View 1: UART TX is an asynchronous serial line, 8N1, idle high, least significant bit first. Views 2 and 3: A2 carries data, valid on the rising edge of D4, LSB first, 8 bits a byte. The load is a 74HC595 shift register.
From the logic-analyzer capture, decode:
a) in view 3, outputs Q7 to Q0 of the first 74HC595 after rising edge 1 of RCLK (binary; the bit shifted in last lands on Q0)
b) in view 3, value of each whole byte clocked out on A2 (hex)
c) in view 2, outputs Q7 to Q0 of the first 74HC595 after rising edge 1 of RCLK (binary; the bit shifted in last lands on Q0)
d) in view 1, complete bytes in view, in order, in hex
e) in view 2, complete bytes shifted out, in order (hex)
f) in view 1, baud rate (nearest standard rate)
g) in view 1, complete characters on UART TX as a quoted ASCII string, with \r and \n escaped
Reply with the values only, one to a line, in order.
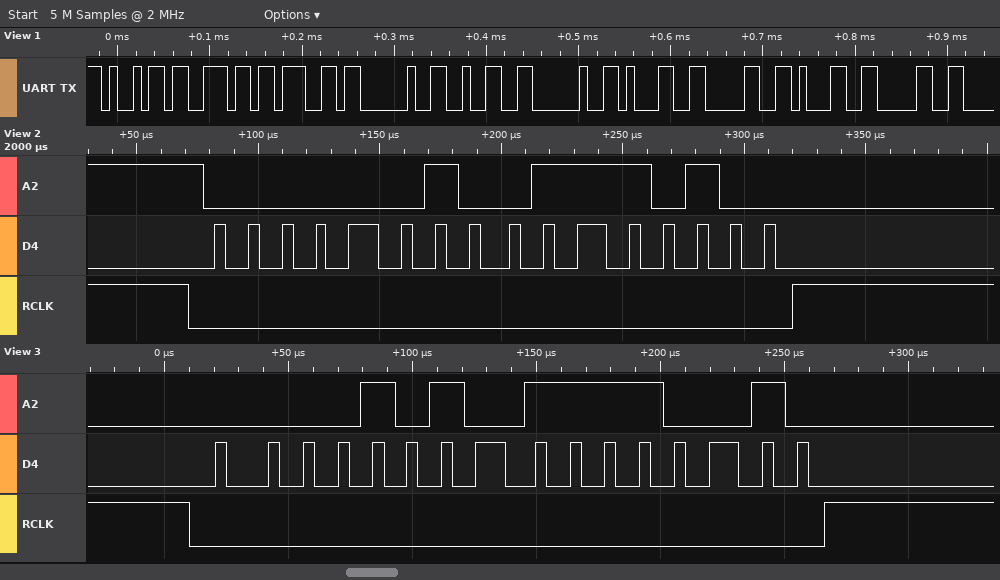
11110010
50 4F
01110100
0x69 0x6E 0x67 0x20 0x32 0x20 0x31 0x30 0x31 0x30
0x40 0x2E
115200 baud
"ing 2 1010"
